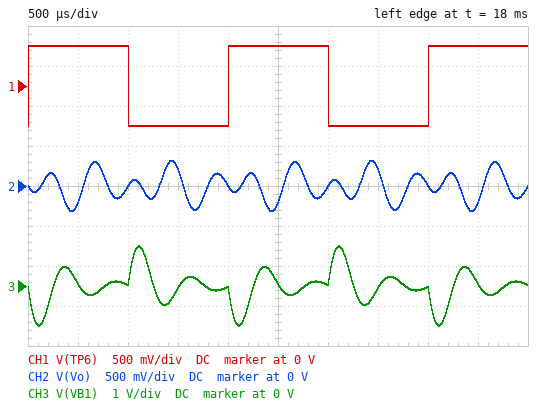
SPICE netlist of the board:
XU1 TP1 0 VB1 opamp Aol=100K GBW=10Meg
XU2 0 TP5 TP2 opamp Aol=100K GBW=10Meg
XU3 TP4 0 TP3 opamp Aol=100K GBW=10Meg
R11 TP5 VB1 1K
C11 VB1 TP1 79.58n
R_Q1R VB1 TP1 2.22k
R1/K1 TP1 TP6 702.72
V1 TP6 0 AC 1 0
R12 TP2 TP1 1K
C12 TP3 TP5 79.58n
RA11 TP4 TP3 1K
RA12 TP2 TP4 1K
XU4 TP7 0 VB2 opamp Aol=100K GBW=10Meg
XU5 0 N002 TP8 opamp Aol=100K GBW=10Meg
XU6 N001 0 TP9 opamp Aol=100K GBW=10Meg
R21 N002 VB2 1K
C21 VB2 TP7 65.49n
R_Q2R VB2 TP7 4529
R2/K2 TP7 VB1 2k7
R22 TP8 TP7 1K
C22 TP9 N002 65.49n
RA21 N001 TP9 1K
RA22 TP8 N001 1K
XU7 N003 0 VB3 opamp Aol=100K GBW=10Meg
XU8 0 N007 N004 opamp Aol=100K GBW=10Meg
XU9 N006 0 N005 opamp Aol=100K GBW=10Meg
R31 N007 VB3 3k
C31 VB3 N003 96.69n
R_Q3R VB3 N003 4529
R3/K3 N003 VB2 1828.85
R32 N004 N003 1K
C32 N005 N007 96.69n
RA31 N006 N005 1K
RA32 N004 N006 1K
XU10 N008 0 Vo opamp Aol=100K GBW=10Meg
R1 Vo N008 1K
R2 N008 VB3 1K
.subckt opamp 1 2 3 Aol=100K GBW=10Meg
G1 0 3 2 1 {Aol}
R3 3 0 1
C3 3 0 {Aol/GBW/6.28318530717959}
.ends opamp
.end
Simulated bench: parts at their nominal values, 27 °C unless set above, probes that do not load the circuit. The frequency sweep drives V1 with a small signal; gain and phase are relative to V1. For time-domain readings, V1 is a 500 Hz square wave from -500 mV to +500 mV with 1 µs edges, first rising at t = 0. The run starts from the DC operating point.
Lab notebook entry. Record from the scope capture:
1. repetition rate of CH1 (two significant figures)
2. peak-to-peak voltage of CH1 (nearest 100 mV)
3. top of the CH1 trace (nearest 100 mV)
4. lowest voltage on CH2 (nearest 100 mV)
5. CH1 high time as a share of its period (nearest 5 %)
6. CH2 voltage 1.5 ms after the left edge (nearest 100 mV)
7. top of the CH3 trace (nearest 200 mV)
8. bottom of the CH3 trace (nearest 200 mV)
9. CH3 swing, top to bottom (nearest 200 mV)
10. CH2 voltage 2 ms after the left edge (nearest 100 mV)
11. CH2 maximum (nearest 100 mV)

500 Hz
1.0 V
500 mV
-300 mV
50 %
200 mV
1.0 V
-1.0 V
2.0 V
0 V
300 mV
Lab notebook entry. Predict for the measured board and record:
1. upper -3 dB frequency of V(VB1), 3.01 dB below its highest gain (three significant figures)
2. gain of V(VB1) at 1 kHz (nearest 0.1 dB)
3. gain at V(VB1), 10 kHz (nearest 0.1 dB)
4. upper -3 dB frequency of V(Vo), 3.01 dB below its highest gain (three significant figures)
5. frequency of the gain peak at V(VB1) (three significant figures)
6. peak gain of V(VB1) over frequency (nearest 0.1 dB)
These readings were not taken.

2.50 kHz
-0.8 dB
-10.6 dB
2.55 kHz
2.00 kHz
10.0 dB
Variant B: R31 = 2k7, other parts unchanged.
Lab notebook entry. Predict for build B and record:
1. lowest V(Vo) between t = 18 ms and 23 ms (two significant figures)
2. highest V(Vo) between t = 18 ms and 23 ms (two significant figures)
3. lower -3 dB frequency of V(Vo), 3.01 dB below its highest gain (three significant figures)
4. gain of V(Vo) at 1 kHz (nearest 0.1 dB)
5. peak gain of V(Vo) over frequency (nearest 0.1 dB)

-330 mV
330 mV
1.91 kHz
-7.7 dB
5.6 dB
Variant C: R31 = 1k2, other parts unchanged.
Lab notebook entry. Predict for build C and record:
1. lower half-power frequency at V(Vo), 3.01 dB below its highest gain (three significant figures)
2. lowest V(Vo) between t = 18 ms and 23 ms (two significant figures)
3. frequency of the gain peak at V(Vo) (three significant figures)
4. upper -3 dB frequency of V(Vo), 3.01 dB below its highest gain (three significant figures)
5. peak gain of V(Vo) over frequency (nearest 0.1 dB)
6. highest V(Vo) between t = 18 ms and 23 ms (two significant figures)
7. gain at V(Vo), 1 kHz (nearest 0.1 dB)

1.54 kHz
-580 mV
2.25 kHz
2.52 kHz
8.5 dB
580 mV
-18.9 dB
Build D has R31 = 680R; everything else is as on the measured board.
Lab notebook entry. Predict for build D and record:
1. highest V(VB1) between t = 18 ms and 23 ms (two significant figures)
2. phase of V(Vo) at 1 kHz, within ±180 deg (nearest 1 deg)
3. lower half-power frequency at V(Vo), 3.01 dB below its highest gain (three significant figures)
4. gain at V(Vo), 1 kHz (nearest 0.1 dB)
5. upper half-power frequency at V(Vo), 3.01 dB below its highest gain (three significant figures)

990 mV
-120 deg
1.91 kHz
-26.1 dB
2.36 kHz
